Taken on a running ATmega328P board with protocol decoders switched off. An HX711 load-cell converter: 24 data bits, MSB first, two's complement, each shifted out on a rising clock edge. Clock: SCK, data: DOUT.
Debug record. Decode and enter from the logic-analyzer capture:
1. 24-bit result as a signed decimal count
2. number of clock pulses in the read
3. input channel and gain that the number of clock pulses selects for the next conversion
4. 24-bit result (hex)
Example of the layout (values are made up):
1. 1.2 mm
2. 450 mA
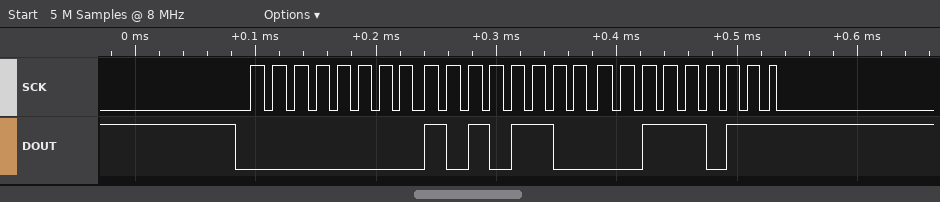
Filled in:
1. 44091
2. 25
3. channel A, gain 128
4. 0x00AC3B
